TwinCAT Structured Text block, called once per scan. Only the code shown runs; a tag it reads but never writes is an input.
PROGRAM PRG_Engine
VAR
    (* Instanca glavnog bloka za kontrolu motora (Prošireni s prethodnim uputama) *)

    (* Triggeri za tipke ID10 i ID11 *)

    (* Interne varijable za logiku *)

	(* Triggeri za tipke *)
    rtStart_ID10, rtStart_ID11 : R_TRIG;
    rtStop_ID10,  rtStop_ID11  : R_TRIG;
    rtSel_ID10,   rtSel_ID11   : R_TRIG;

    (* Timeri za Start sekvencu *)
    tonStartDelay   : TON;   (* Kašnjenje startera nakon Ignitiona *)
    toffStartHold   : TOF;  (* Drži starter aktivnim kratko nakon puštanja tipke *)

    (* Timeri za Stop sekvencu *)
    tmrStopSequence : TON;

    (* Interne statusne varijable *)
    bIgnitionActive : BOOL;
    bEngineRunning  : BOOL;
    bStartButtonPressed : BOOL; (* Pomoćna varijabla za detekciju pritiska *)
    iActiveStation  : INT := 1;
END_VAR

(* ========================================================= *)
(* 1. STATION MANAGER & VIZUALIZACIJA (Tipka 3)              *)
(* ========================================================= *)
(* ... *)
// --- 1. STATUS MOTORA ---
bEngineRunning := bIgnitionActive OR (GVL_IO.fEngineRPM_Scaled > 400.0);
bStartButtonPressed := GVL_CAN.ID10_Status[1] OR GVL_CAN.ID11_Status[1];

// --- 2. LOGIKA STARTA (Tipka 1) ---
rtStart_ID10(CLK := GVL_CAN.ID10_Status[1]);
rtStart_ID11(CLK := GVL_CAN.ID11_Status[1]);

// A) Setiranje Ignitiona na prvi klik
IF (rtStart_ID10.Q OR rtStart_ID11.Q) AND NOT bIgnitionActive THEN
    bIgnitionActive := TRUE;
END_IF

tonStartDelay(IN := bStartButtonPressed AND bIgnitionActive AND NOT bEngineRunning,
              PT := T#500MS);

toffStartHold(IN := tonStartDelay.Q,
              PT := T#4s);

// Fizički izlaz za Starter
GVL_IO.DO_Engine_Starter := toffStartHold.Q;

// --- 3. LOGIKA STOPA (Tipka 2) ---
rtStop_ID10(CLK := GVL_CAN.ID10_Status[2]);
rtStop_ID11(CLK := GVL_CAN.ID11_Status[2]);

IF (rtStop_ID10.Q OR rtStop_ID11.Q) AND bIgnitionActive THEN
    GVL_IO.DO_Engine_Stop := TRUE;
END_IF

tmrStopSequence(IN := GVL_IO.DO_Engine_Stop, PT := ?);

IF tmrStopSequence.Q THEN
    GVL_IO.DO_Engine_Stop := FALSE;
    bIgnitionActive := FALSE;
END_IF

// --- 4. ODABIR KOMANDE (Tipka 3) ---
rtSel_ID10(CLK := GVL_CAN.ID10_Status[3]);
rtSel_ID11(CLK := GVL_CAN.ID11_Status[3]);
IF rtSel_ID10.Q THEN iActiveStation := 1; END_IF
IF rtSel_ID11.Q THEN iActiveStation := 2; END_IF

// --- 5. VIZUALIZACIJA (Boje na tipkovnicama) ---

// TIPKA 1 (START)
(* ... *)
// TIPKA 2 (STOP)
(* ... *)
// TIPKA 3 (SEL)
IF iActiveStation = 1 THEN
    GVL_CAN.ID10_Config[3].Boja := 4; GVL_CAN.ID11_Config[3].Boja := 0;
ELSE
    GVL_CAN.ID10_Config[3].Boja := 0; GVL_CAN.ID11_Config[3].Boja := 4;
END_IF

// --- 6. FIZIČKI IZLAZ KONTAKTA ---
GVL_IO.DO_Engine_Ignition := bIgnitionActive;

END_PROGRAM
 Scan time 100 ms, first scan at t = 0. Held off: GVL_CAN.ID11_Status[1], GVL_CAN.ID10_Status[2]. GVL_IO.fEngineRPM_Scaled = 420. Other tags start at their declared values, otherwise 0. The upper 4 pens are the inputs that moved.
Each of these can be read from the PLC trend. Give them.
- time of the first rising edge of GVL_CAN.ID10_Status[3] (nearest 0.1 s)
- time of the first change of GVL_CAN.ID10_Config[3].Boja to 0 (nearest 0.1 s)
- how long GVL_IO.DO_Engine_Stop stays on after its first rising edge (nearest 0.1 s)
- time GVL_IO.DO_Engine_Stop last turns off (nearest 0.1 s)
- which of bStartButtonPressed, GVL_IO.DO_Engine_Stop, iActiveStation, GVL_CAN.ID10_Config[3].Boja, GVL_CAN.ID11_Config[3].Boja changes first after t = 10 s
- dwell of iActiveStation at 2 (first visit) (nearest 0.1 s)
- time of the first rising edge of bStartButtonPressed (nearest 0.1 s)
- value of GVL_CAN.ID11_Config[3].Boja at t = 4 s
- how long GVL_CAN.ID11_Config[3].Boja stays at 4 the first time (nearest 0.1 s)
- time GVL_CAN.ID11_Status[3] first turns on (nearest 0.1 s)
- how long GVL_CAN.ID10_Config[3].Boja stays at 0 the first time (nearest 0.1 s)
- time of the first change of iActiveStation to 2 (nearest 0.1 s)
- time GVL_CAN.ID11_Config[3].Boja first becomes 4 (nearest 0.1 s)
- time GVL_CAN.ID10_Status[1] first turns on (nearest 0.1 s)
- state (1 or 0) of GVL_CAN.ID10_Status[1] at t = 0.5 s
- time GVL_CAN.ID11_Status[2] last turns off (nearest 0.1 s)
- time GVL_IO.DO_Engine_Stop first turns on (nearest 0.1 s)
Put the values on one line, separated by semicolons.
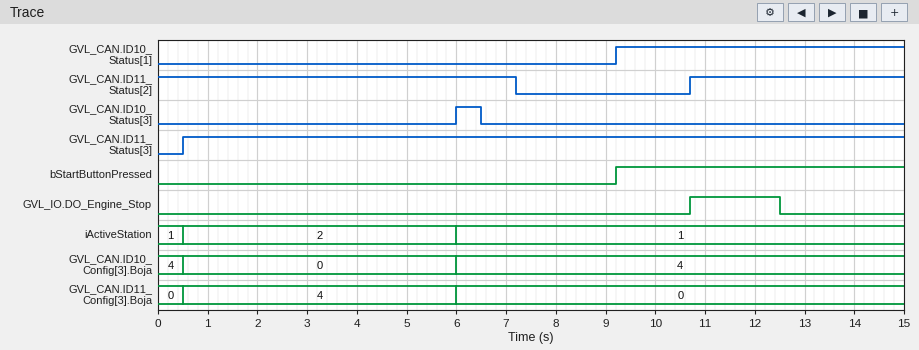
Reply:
6.0 s; 0.5 s; 1.8 s; 12.5 s; GVL_IO.DO_Engine_Stop; 5.5 s; 9.2 s; 4; 5.5 s; 0.5 s; 5.5 s; 0.5 s; 0.5 s; 9.2 s; 0; 7.2 s; 10.7 s
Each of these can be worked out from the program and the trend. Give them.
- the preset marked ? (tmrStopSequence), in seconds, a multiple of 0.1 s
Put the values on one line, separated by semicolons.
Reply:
1.8 s
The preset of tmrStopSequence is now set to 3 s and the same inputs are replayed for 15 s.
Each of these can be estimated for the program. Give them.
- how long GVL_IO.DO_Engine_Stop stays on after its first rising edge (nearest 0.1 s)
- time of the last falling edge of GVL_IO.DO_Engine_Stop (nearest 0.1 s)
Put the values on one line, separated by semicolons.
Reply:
3.0 s; 13.7 s
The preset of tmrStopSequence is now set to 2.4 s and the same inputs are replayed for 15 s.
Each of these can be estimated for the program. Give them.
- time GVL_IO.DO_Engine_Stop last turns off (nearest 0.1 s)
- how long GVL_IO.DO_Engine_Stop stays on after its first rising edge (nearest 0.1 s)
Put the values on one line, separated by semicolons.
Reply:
13.1 s; 2.4 s
